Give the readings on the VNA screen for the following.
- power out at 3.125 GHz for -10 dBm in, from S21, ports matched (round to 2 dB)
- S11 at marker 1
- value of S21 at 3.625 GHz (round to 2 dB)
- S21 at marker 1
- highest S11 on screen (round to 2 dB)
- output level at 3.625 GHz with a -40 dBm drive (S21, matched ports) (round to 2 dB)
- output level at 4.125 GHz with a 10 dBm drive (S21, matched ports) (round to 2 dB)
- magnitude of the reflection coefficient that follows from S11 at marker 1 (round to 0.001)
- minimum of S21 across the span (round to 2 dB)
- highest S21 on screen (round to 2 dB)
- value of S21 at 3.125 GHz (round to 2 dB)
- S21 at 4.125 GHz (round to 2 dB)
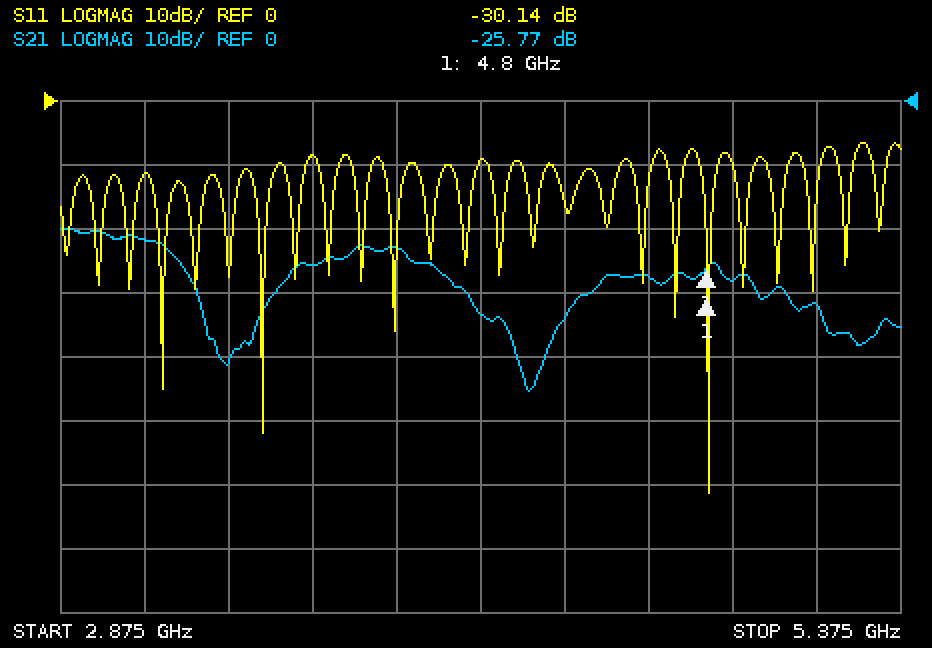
-32 dBm
-30.14 dB
-26 dB
-25.77 dB
-6 dB
-66 dBm
-24 dBm
0.031
-46 dB
-20 dB
-22 dB
-34 dB
